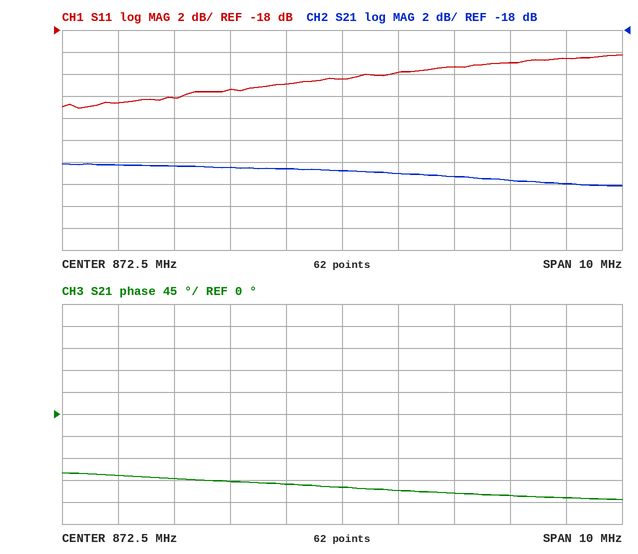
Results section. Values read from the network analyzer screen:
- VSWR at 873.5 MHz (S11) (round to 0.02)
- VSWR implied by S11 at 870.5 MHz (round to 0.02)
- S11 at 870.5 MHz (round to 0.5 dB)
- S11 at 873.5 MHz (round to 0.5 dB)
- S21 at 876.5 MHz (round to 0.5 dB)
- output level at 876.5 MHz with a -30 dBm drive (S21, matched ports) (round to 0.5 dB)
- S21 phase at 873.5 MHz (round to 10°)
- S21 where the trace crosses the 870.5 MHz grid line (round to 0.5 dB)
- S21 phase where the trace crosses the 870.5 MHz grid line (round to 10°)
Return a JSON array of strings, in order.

["1.18", "1.14", "-23.5 dB", "-22.0 dB", "-32.0 dB", "-62.0 dBm", "-160°", "-30.5 dB", "-140°"]
